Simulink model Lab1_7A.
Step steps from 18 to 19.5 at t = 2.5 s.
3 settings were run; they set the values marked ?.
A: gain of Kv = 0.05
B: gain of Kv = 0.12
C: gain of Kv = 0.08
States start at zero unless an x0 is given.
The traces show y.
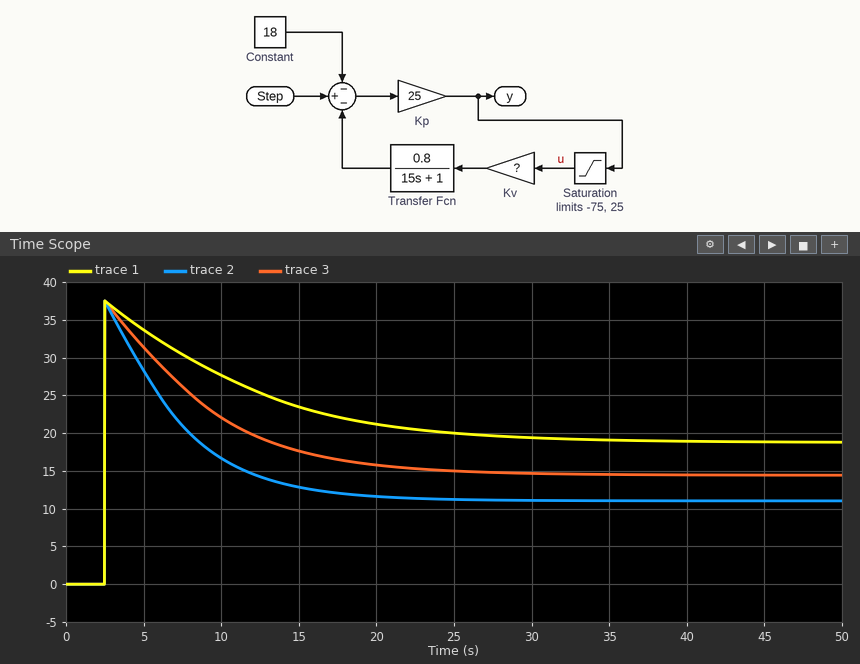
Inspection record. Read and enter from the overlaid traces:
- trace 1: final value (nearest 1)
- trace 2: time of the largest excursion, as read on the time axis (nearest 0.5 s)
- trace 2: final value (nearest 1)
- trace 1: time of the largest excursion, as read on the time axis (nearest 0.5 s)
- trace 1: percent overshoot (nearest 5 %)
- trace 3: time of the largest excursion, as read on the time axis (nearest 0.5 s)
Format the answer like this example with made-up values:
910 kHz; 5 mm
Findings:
19; 2.5 s; 11; 2.5 s; 100 %; 2.5 s
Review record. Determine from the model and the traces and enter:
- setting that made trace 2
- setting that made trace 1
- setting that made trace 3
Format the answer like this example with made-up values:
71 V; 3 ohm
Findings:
B; A; C
